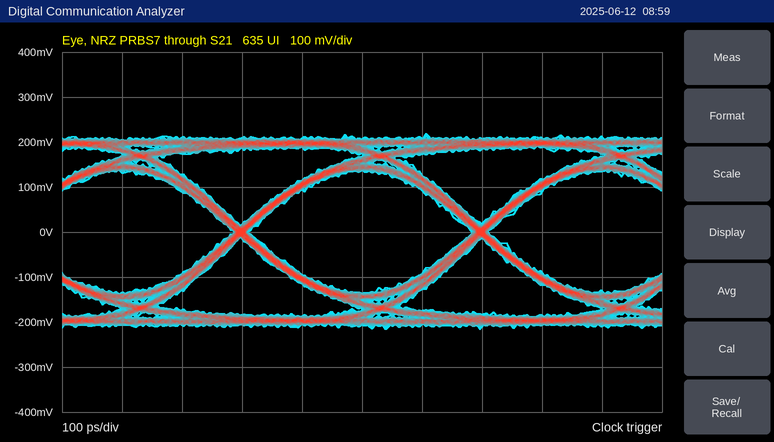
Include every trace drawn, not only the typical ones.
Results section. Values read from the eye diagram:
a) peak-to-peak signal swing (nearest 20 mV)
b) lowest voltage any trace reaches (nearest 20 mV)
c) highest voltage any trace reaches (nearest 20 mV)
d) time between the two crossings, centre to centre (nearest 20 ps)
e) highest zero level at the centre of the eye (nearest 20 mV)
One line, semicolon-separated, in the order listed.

440 mV; -220 mV; 220 mV; 400 ps; -140 mV
